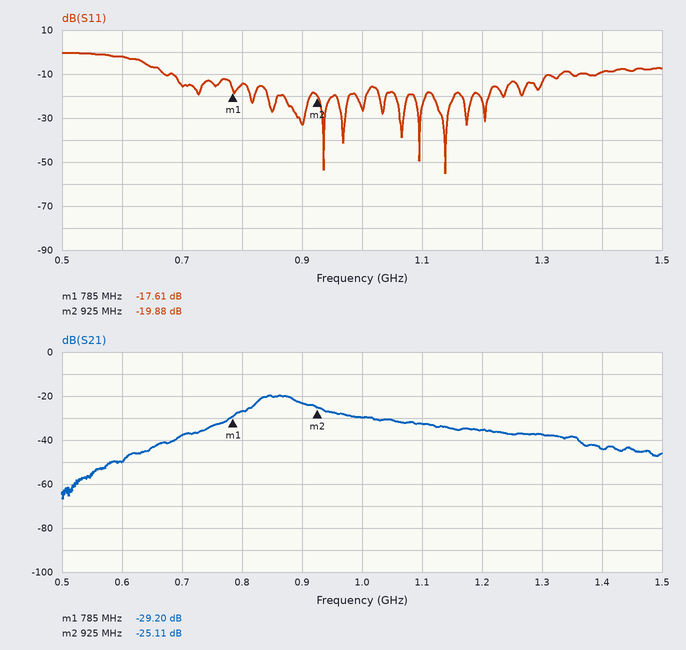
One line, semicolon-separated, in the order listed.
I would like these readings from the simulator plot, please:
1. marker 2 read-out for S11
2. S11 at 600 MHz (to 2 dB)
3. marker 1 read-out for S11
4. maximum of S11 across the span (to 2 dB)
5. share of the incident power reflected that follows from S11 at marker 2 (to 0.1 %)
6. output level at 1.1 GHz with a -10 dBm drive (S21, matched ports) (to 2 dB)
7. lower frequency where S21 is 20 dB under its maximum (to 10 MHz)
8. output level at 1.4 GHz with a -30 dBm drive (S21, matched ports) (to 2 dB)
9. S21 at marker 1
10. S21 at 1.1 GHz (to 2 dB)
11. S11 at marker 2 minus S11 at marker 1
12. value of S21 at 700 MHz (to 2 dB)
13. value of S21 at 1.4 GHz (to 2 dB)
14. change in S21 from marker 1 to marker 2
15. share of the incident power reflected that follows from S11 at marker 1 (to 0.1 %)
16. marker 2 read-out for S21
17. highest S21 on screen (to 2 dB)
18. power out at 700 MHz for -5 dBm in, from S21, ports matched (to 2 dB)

-19.88 dB; -2 dB; -17.61 dB; 0 dB; 1.0 %; -42 dBm; 690 MHz; -74 dBm; -29.20 dB; -32 dB; -2.27 dB; -38 dB; -44 dB; 4.09 dB; 1.7 %; -25.11 dB; -20 dB; -42 dBm
